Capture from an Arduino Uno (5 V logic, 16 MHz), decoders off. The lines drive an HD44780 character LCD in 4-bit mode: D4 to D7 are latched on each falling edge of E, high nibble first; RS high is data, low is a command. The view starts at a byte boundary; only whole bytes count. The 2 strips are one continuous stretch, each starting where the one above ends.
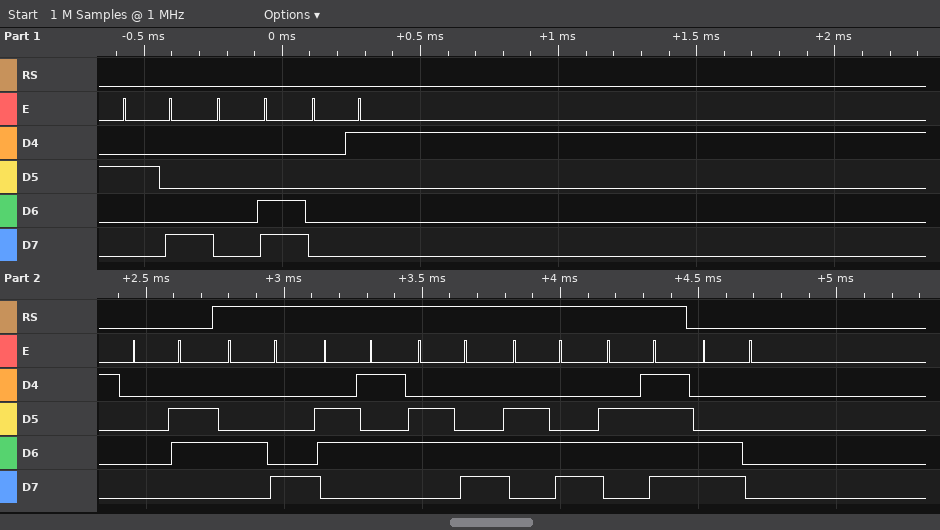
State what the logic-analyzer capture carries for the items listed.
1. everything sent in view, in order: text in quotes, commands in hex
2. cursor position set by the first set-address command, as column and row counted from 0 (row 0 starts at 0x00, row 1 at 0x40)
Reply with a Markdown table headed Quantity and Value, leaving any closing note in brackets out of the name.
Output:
| Quantity | Value |
|---|---|
| everything sent in view, in order: text in quotes, commands in hex | 0x28 0x0C 0x01 0x06 "Hello" 0xC0 |
| cursor position set by the first set-address command, as column and row counted from 0 | column 0, row 1 |
